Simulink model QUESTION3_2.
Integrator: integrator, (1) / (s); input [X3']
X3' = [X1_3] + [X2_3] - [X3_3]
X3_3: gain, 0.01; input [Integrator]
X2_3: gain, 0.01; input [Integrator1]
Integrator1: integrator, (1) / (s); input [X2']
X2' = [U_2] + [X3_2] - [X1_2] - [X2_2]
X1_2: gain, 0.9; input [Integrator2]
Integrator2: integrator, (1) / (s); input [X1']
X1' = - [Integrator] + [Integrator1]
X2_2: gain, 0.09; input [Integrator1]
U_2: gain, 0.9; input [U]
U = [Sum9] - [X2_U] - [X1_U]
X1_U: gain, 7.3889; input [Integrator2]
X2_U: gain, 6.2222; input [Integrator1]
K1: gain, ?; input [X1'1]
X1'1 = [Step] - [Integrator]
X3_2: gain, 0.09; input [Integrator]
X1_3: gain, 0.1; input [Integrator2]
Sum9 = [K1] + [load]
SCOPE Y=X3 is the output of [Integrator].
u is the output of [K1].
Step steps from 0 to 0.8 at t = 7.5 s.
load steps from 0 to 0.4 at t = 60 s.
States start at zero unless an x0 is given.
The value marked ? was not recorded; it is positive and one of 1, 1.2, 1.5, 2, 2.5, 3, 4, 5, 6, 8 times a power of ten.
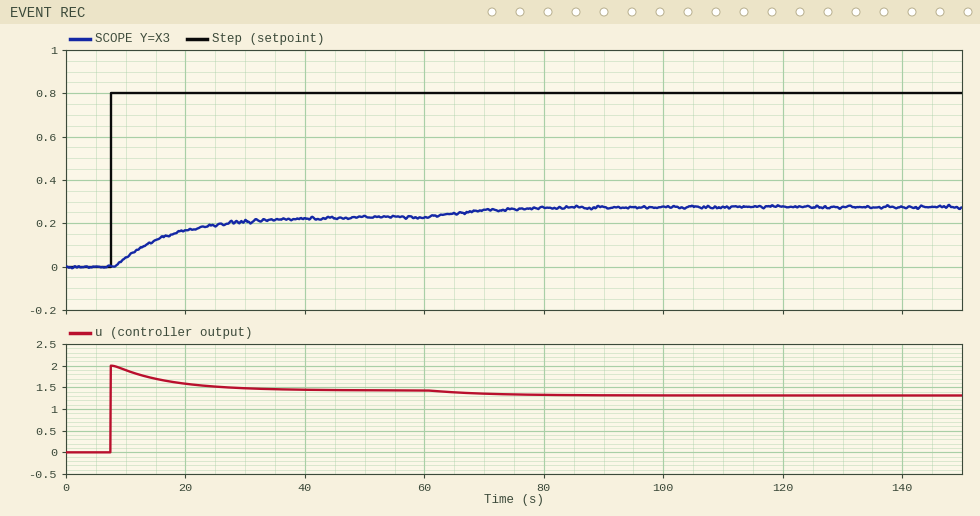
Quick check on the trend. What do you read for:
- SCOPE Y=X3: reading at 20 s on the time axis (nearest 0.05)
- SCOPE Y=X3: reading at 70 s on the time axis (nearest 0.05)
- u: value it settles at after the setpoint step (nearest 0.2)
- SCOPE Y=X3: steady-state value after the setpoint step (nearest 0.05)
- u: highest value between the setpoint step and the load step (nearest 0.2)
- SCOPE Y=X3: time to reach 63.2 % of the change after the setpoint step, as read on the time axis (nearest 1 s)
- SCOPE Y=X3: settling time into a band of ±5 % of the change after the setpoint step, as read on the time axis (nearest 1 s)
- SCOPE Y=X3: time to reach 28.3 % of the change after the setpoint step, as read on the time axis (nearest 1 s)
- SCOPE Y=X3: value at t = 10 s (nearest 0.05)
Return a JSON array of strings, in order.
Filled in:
["0.15", "0.25", "1.4", "0.25", "2.0", "17 s", "35 s", "11 s", "0.05"]
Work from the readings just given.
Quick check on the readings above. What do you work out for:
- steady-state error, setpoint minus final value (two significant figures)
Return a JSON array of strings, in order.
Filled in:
["0.55"]
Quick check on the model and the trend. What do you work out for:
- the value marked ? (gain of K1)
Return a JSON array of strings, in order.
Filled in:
["2.5"]
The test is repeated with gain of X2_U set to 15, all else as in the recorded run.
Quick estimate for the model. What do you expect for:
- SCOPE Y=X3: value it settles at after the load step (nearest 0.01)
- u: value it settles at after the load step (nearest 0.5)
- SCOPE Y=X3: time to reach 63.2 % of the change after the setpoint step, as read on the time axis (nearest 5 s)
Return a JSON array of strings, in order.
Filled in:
["0.14", "1.5", "15 s"]
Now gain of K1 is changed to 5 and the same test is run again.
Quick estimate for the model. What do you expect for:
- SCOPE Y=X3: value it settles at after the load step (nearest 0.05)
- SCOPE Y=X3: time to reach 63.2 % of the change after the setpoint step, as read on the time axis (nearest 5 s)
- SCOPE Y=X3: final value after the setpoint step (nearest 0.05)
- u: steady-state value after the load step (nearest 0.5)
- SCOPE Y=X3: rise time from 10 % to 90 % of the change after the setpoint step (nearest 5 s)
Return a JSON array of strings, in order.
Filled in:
["0.40", "15 s", "0.35", "2.0", "15 s"]
